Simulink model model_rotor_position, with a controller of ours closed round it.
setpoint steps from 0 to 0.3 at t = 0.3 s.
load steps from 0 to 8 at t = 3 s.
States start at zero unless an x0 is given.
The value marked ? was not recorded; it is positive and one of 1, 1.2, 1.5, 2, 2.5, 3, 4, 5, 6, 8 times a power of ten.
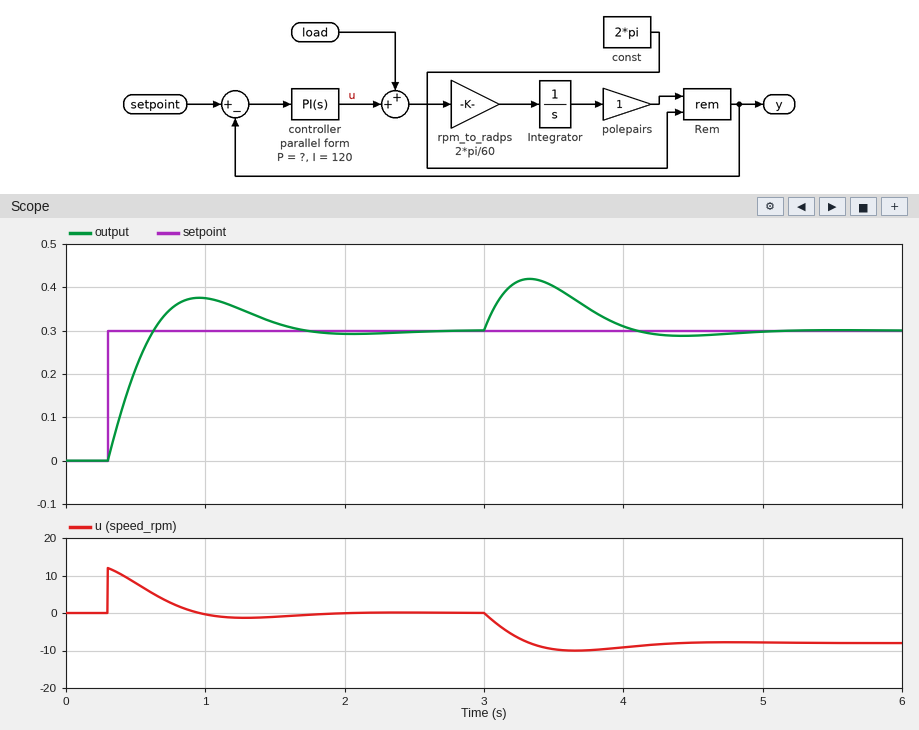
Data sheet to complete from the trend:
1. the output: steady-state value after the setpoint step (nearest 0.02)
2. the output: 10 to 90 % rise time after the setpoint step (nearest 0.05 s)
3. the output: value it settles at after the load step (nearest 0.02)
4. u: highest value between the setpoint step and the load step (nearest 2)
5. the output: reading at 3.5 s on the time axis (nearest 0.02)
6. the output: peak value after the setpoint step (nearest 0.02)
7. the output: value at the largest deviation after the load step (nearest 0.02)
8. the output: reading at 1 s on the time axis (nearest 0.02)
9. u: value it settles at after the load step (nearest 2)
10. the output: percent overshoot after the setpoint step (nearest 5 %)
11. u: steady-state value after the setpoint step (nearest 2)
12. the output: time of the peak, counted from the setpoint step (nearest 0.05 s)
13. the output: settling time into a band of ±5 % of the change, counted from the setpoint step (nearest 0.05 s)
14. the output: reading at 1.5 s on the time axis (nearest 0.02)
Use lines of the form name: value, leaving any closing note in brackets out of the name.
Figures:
the output: steady-state value after the setpoint step: 0.30
the output: 10 to 90 % rise time after the setpoint step: 0.25 s
the output: value it settles at after the load step: 0.30
u: highest value between the setpoint step and the load step: 12
the output: reading at 3.5 s on the time axis: 0.40
the output: peak value after the setpoint step: 0.38
the output: value at the largest deviation after the load step: 0.42
the output: reading at 1 s on the time axis: 0.38
u: value it settles at after the load step: -8
the output: percent overshoot after the setpoint step: 25 %
u: steady-state value after the setpoint step: 0
the output: time of the peak, counted from the setpoint step: 0.65 s
the output: settling time into a band of ±5 % of the change, counted from the setpoint step: 1.25 s
the output: reading at 1.5 s on the time axis: 0.32
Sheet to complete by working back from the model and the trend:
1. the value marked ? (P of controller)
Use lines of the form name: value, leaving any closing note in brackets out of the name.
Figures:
the value marked ?: 40
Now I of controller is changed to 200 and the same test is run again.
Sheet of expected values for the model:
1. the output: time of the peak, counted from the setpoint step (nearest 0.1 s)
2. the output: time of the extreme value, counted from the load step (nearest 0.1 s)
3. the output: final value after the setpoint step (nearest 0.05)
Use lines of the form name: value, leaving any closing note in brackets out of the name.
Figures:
the output: time of the peak, counted from the setpoint step: 0.5 s
the output: time of the extreme value, counted from the load step: 0.3 s
the output: final value after the setpoint step: 0.30
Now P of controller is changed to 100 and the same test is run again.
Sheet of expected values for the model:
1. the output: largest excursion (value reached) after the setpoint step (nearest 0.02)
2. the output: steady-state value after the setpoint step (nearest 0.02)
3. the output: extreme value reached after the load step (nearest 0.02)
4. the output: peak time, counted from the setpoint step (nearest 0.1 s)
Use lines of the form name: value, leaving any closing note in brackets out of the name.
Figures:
the output: largest excursion (value reached) after the setpoint step: 0.32
the output: steady-state value after the setpoint step: 0.30
the output: extreme value reached after the load step: 0.36
the output: peak time, counted from the setpoint step: 0.5 s
